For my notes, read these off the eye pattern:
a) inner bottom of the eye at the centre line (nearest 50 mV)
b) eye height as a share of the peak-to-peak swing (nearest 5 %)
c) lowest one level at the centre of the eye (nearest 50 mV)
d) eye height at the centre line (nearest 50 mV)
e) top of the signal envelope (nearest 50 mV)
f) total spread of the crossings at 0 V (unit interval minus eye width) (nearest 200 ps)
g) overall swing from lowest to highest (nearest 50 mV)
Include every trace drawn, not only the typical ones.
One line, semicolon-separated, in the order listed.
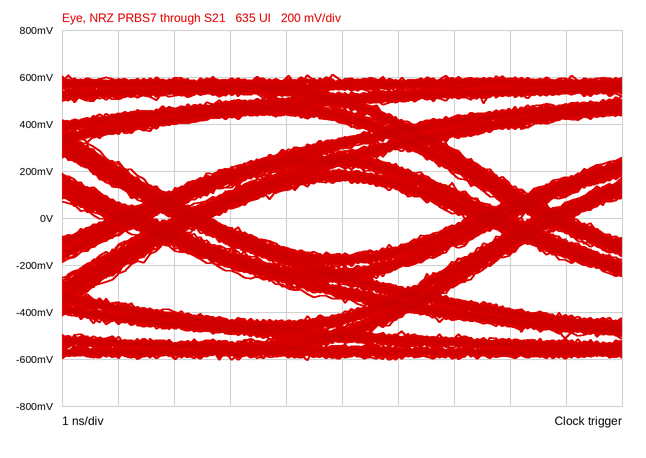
-150 mV; 25 %; 150 mV; 300 mV; 600 mV; 2.0 ns; 1.20 V
